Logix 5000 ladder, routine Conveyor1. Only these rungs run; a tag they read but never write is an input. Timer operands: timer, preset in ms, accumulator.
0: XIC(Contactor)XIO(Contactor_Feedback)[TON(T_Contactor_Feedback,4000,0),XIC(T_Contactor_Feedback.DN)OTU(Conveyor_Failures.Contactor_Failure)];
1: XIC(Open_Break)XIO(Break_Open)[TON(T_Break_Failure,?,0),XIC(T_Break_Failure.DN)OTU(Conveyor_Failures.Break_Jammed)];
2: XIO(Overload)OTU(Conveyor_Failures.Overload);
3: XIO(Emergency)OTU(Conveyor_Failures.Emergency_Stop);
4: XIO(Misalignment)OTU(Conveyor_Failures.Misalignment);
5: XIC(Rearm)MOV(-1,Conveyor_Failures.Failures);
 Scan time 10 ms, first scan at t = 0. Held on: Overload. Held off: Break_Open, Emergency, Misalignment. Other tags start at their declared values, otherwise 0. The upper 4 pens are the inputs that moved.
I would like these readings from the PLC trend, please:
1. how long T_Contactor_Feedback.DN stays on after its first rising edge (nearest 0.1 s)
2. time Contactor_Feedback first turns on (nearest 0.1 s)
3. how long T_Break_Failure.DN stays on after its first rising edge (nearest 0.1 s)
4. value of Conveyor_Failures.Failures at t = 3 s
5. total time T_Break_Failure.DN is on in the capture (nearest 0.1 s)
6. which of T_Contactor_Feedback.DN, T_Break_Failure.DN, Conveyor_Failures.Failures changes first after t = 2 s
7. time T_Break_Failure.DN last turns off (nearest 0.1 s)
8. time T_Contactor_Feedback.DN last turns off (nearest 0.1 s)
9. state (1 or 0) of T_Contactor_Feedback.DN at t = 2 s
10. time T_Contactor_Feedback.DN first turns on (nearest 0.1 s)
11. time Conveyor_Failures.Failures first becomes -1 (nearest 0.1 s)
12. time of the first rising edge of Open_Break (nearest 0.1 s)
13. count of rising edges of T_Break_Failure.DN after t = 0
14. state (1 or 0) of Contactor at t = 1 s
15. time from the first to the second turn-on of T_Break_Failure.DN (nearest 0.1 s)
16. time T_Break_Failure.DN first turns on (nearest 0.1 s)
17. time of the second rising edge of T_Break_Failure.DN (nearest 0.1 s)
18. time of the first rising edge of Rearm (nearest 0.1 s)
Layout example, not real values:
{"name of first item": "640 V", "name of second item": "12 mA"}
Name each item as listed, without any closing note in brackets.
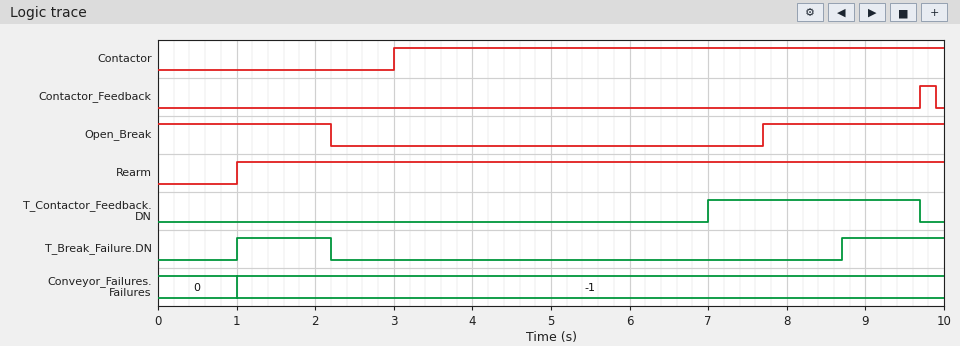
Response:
{"how long T_Contactor_Feedback.DN stays on after its first rising edge": "2.7 s", "time Contactor_Feedback first turns on": "9.7 s", "how long T_Break_Failure.DN stays on after its first rising edge": "1.2 s", "value of Conveyor_Failures.Failures at t = 3 s": "-1", "total time T_Break_Failure.DN is on in the capture": "2.5 s", "which of T_Contactor_Feedback.DN, T_Break_Failure.DN, Conveyor_Failures.Failures changes first after t = 2 s": "T_Break_Failure.DN", "time T_Break_Failure.DN last turns off": "2.2 s", "time T_Contactor_Feedback.DN last turns off": "9.7 s", "state (1 or 0) of T_Contactor_Feedback.DN at t = 2 s": "0", "time T_Contactor_Feedback.DN first turns on": "7.0 s", "time Conveyor_Failures.Failures first becomes -1": "1.0 s", "time of the first rising edge of Open_Break": "7.7 s", "count of rising edges of T_Break_Failure.DN after t = 0": "2", "state (1 or 0) of Contactor at t = 1 s": "0", "time from the first to the second turn-on of T_Break_Failure.DN": "7.7 s", "time T_Break_Failure.DN first turns on": "1.0 s", "time of the second rising edge of T_Break_Failure.DN": "8.7 s", "time of the first rising edge of Rearm": "1.0 s"}
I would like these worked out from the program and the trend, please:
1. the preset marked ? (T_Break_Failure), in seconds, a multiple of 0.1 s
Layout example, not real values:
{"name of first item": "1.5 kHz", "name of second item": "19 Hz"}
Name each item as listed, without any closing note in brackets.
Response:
{"the preset marked ? (T_Break_Failure), in seconds, a multiple of 0.1 s": "1.0 s"}
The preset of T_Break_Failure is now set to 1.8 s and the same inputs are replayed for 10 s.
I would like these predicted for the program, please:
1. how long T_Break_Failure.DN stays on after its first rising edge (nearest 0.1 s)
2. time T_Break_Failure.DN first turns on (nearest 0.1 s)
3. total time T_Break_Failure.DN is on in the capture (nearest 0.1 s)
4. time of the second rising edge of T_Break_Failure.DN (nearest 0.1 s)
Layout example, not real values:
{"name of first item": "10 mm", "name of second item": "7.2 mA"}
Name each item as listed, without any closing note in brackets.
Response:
{"how long T_Break_Failure.DN stays on after its first rising edge": "0.4 s", "time T_Break_Failure.DN first turns on": "1.8 s", "total time T_Break_Failure.DN is on in the capture": "0.9 s", "time of the second rising edge of T_Break_Failure.DN": "9.5 s"}
